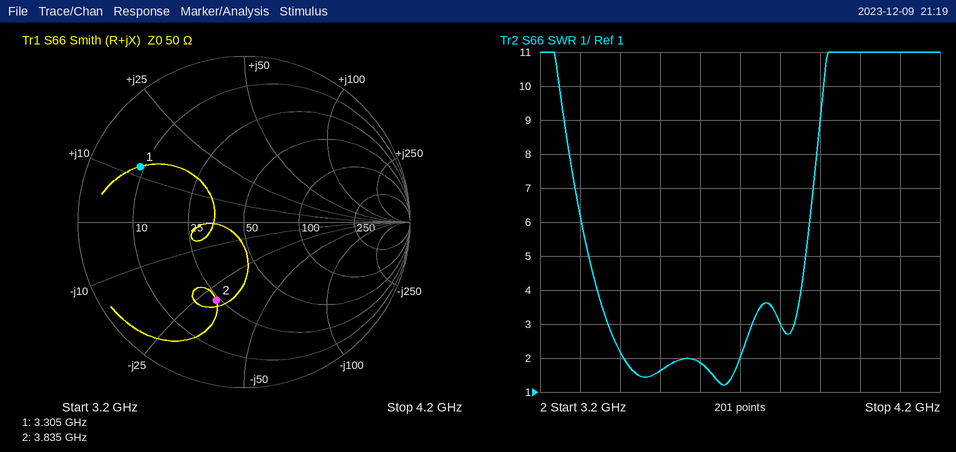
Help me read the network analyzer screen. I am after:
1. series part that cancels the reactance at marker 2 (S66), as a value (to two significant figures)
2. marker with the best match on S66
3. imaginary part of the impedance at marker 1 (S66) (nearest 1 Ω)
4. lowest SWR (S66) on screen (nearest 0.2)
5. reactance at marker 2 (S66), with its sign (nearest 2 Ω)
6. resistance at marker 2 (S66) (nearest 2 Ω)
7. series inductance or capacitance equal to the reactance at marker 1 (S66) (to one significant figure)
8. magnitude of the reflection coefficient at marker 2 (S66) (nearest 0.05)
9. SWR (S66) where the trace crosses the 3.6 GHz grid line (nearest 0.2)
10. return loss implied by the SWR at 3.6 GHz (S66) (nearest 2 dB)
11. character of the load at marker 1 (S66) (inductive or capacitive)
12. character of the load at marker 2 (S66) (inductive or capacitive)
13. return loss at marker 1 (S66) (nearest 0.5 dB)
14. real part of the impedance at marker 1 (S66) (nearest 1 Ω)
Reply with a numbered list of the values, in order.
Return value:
1. 1.2 nH
2. marker 2
3. +12 Ω
4. 1.2
5. -30 Ω
6. 24 Ω
7. 600 pH
8. 0.50
9. 1.8
10. 10 dB
11. inductive
12. capacitive
13. 3.0 dB
14. 9 Ω
